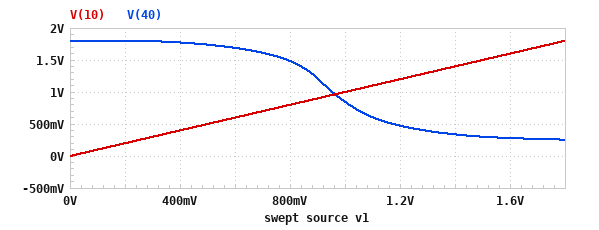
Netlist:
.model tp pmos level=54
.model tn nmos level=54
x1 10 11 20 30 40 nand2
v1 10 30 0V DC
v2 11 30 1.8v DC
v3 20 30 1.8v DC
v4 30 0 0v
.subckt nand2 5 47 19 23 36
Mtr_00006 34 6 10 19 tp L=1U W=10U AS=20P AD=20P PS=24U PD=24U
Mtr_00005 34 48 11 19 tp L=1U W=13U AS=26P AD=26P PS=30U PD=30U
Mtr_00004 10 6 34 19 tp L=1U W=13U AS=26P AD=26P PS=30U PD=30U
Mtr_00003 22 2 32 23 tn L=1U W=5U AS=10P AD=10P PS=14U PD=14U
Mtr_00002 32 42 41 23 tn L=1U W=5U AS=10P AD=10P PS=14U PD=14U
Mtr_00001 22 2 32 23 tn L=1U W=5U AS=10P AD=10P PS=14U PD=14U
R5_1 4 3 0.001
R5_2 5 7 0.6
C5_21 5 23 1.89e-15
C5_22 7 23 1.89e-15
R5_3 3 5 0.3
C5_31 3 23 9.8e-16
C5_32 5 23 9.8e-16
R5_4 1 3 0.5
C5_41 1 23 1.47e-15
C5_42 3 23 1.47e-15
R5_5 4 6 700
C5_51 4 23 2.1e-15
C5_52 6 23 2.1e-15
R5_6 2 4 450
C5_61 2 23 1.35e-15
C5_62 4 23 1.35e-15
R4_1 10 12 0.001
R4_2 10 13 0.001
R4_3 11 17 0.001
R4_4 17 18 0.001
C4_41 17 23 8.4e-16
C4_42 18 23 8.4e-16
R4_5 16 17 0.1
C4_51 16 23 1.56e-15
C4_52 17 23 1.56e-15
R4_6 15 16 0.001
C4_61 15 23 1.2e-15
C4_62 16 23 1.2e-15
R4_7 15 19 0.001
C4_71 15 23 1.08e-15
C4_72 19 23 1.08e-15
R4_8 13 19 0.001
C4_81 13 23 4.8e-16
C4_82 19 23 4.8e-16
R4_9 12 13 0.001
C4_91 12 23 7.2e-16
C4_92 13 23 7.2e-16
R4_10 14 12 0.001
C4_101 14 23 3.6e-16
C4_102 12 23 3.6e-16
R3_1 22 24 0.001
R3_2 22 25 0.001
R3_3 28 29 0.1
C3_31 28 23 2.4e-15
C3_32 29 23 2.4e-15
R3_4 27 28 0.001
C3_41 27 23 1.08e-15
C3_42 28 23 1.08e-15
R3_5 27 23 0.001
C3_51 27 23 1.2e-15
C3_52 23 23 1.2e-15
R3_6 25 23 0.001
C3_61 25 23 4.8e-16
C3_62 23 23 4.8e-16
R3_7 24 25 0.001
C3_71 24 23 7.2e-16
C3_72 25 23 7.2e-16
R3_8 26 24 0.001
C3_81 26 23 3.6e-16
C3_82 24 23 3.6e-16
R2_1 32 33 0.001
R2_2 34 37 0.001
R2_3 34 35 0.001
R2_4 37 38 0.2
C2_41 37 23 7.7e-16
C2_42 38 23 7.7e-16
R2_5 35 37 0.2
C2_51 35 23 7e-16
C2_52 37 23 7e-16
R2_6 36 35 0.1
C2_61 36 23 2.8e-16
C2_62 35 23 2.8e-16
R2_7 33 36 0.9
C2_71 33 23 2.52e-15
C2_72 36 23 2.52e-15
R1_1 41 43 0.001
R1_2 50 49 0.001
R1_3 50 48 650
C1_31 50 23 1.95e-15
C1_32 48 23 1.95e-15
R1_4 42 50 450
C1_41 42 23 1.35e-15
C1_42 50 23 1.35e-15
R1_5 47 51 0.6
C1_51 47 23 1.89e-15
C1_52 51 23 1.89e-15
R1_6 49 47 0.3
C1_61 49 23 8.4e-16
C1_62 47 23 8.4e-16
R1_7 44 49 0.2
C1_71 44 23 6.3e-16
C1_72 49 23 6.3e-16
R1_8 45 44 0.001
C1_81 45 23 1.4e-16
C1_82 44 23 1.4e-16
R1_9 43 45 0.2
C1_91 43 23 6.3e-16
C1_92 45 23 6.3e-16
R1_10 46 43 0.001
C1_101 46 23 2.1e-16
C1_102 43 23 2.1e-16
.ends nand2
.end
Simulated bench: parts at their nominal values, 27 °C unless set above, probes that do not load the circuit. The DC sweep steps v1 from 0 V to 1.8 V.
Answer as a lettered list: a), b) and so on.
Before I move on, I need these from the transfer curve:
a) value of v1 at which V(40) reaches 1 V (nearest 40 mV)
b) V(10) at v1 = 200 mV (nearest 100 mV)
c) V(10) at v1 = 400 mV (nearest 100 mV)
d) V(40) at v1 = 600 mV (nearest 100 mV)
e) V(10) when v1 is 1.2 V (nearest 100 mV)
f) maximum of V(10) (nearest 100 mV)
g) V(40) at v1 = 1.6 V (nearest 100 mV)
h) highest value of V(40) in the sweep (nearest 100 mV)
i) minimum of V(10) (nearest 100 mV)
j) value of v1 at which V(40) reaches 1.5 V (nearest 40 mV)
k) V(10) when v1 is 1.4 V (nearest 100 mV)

a) 960 mV
b) 200 mV
c) 400 mV
d) 1.7 V
e) 1.2 V
f) 1.8 V
g) 300 mV
h) 1.8 V
i) 0 V
j) 800 mV
k) 1.4 V
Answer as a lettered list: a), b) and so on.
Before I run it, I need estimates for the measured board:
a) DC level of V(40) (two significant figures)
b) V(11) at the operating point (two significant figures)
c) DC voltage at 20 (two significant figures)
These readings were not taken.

a) 1.8 V
b) 1.8 V
c) 1.8 V
